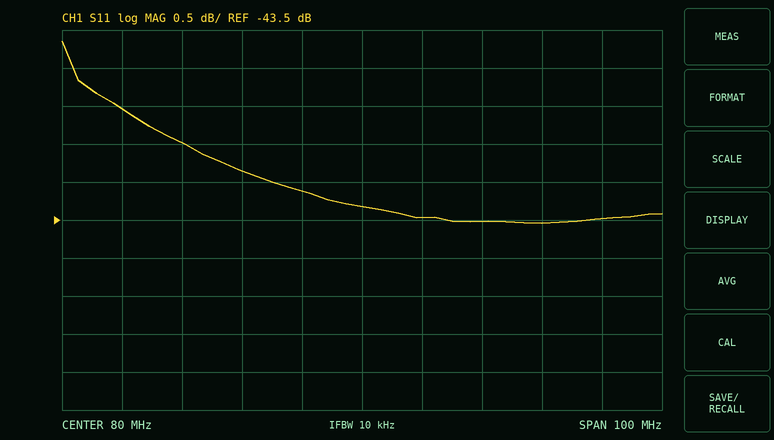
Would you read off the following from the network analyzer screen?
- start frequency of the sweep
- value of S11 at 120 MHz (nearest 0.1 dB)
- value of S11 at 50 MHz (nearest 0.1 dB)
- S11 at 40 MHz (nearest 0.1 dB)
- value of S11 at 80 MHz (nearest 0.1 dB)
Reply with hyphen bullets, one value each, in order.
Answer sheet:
- 30 MHz
- -43.5 dB
- -42.5 dB
- -42.0 dB
- -43.3 dB
